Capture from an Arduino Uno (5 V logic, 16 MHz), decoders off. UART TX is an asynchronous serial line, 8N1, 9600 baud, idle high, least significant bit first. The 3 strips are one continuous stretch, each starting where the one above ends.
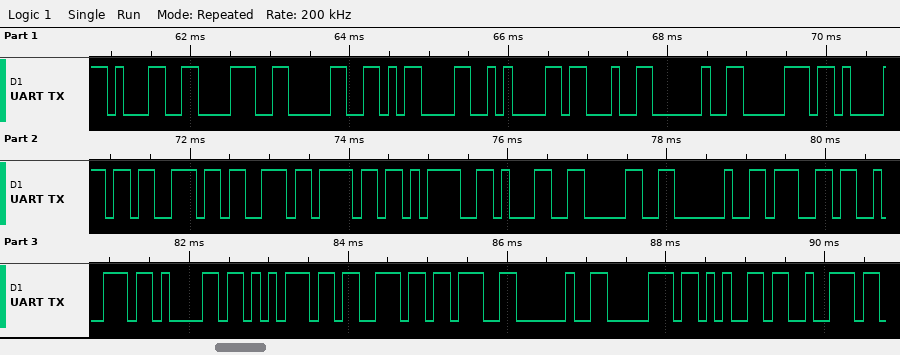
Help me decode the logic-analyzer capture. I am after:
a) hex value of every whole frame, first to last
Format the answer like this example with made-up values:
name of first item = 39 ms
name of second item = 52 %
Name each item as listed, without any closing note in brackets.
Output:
hex value of every whole frame, first to last = 31 38 30 0D 0A 23 20 70 61 73 73 6F 3D 31 30 20 67 72 61 75 73 3B 20 70 65 72
